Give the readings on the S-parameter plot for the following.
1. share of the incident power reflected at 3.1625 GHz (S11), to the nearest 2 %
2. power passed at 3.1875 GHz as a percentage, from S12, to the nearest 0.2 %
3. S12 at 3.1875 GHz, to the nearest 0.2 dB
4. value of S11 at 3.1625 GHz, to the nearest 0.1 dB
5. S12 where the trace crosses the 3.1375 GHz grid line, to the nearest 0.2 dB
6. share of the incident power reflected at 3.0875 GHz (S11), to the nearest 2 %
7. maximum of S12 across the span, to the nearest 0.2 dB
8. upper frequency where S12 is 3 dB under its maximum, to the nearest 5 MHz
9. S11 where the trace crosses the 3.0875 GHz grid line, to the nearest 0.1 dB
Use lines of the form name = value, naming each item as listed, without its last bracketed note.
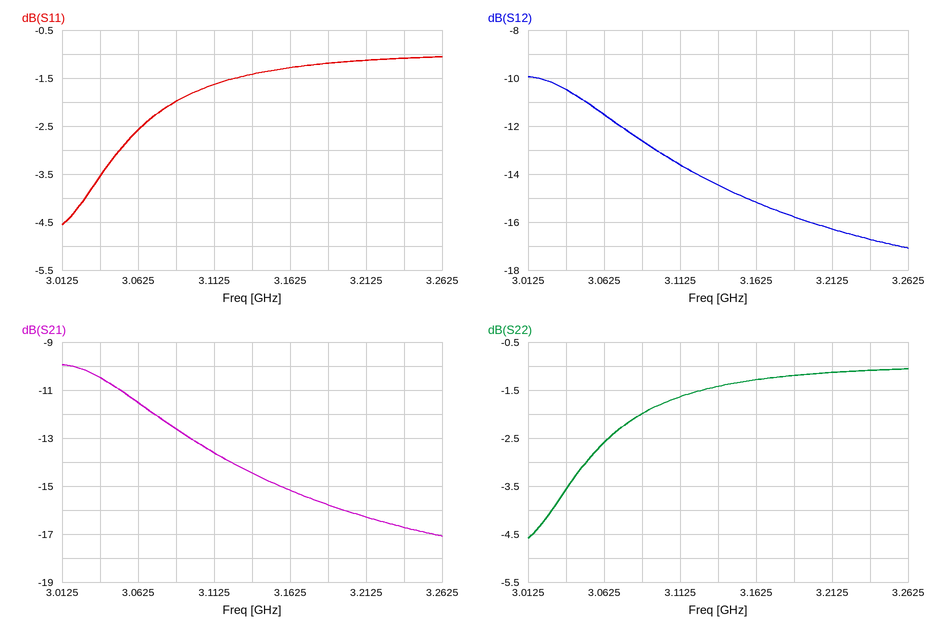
share of the incident power reflected at 3.1625 GHz (S11), to the nearest 2 % = 74 %
power passed at 3.1875 GHz as a percentage, from S12, to the nearest 0.2 % = 2.6 %
S12 at 3.1875 GHz, to the nearest 0.2 dB = -15.8 dB
value of S11 at 3.1625 GHz, to the nearest 0.1 dB = -1.3 dB
S12 where the trace crosses the 3.1375 GHz grid line, to the nearest 0.2 dB = -14.4 dB
share of the incident power reflected at 3.0875 GHz (S11), to the nearest 2 % = 64 %
maximum of S12 across the span, to the nearest 0.2 dB = -10.0 dB
upper frequency where S12 is 3 dB under its maximum, to the nearest 5 MHz = 3.095 GHz
S11 where the trace crosses the 3.0875 GHz grid line, to the nearest 0.1 dB = -2.0 dB
